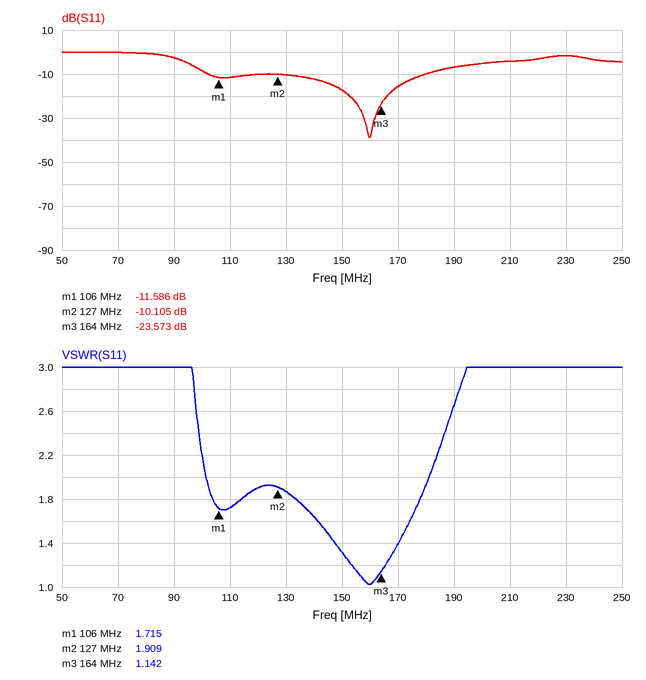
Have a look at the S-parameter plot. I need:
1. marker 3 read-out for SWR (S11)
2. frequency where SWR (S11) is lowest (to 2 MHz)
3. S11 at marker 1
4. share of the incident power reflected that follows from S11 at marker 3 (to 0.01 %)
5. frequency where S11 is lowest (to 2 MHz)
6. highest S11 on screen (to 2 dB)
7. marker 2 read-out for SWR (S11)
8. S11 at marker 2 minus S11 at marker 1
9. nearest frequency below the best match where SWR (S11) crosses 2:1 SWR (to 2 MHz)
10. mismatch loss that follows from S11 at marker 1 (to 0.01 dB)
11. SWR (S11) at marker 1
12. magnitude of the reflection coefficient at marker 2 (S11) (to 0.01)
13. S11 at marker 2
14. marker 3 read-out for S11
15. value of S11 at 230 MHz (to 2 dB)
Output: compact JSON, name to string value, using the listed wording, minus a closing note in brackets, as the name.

{"marker 3 read-out for SWR": "1.142", "frequency where SWR (S11) is lowest": "160 MHz", "S11 at marker 1": "-11.586 dB", "share of the incident power reflected that follows from S11 at marker 3": "0.44 %", "frequency where S11 is lowest": "160 MHz", "highest S11 on screen": "0 dB", "marker 2 read-out for SWR": "1.909", "S11 at marker 2 minus S11 at marker 1": "1.481 dB", "nearest frequency below the best match where SWR (S11) crosses 2:1 SWR": "102 MHz", "mismatch loss that follows from S11 at marker 1": "0.31 dB", "SWR (S11) at marker 1": "1.715", "magnitude of the reflection coefficient at marker 2 (S11)": "0.31", "S11 at marker 2": "-10.105 dB", "marker 3 read-out for S11": "-23.573 dB", "value of S11 at 230 MHz": "-2 dB"}
